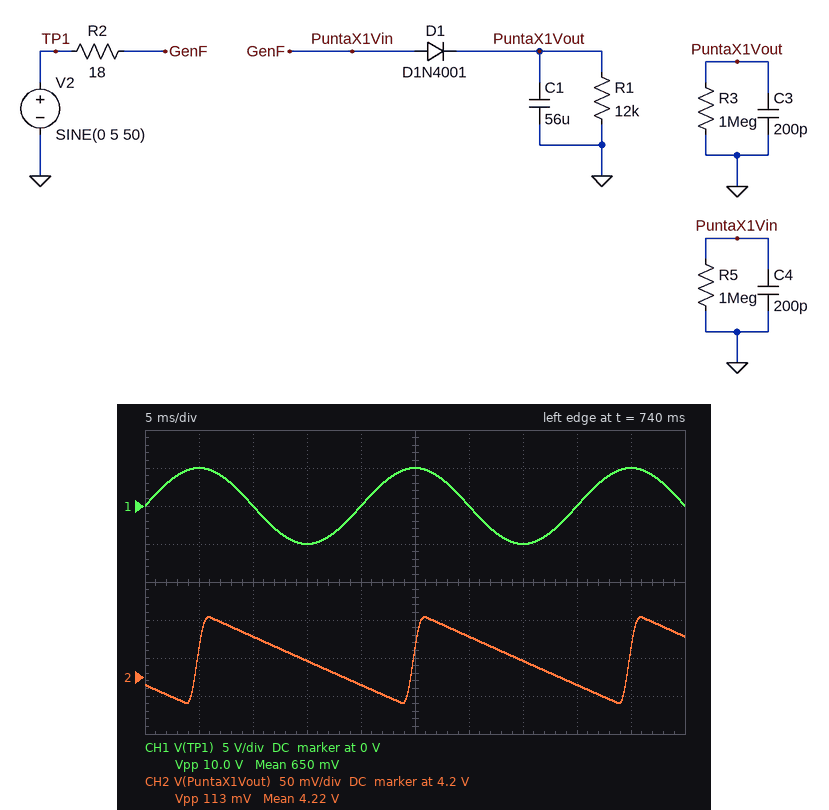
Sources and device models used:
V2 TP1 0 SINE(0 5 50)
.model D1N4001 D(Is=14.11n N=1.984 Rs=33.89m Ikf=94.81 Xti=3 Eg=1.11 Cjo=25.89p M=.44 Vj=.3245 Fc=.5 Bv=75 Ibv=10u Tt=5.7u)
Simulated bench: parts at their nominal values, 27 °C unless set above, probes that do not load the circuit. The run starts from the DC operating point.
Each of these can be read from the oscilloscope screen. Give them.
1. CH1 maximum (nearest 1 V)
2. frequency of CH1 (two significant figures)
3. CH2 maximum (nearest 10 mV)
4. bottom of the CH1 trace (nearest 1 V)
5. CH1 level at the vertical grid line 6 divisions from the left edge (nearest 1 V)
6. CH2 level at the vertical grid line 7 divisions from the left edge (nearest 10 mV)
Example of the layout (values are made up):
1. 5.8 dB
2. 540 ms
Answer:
1. 5 V
2. 50 Hz
3. 4.28 V
4. -5 V
5. 0 V
6. 4.22 V
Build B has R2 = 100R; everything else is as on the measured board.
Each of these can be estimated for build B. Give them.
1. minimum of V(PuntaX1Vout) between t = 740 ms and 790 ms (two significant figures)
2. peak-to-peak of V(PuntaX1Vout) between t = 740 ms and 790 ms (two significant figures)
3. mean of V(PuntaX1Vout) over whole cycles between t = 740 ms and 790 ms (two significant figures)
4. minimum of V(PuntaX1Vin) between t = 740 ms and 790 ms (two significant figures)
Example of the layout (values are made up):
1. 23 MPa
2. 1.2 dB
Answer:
1. 3.9 V
2. 100 mV
3. 4.0 V
4. -5.0 V
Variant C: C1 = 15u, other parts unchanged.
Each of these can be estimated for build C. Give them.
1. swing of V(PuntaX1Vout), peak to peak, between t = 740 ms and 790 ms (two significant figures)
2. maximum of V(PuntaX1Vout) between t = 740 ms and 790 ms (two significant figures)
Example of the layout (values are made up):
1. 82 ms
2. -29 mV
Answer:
1. 410 mV
2. 4.4 V
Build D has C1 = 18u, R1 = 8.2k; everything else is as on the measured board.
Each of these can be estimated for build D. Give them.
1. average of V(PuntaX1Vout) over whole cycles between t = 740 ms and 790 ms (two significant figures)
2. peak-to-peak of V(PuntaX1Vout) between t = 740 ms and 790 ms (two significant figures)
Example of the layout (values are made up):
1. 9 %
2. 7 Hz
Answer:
1. 4.1 V
2. 490 mV
